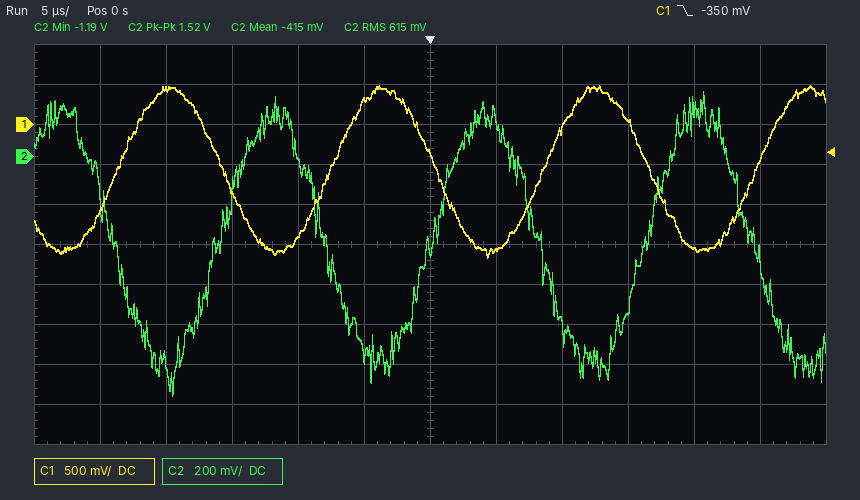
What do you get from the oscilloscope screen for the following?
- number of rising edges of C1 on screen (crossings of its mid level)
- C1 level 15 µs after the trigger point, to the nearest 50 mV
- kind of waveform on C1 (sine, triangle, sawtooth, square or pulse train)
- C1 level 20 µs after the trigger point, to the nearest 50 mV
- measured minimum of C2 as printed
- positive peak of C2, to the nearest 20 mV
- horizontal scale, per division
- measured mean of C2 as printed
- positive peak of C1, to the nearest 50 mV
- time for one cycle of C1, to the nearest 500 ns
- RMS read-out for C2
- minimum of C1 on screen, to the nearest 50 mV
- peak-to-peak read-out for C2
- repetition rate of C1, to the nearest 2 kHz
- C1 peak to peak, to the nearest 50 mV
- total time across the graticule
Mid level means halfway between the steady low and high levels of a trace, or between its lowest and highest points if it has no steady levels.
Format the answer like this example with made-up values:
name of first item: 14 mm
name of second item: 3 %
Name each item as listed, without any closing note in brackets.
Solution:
number of rising edges of C1 on screen: 4
C1 level 15 µs after the trigger point, to the nearest 50 mV: 50 mV
kind of waveform on C1: sine
C1 level 20 µs after the trigger point, to the nearest 50 mV: -1.55 V
measured minimum of C2 as printed: -1.19 V
positive peak of C2, to the nearest 20 mV: 320 mV
horizontal scale, per division: 5 µs
measured mean of C2 as printed: -415 mV
positive peak of C1, to the nearest 50 mV: 500 mV
time for one cycle of C1, to the nearest 500 ns: 16.0 µs
RMS read-out for C2: 615 mV
minimum of C1 on screen, to the nearest 50 mV: -1.65 V
peak-to-peak read-out for C2: 1.52 V
repetition rate of C1, to the nearest 2 kHz: 62 kHz
C1 peak to peak, to the nearest 50 mV: 2.15 V
total time across the graticule: 60 µs
